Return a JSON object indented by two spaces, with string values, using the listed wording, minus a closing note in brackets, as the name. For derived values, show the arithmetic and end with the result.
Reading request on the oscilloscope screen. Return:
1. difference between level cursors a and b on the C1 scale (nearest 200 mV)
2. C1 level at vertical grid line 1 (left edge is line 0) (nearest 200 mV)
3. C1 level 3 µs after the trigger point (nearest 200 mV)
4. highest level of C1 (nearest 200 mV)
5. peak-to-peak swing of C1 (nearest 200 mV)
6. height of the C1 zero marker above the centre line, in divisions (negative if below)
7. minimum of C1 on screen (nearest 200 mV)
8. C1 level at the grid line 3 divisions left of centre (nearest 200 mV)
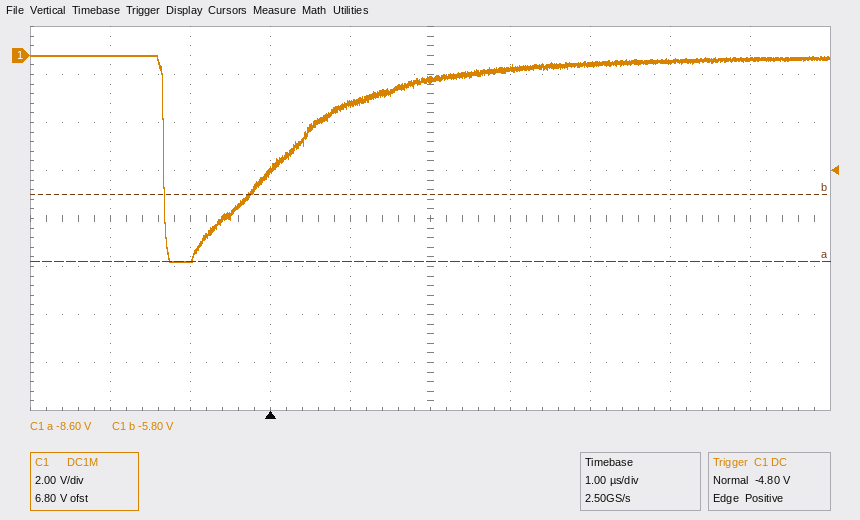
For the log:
{
  "difference between level cursors a and b on the C1 scale": "2.8 V",
  "C1 level at vertical grid line 1 (left edge is line 0)": "0.0 V",
  "C1 level 3 µs after the trigger point": "-600 mV",
  "highest level of C1": "0.0 V",
  "peak-to-peak swing of C1": "0.0 V − (-8.6 V) = 8.6 V",
  "height of the C1 zero marker above the centre line, in divisions": "+3.4 div",
  "minimum of C1 on screen": "-8.6 V",
  "C1 level at the grid line 3 divisions left of centre": "-8.4 V"
}
